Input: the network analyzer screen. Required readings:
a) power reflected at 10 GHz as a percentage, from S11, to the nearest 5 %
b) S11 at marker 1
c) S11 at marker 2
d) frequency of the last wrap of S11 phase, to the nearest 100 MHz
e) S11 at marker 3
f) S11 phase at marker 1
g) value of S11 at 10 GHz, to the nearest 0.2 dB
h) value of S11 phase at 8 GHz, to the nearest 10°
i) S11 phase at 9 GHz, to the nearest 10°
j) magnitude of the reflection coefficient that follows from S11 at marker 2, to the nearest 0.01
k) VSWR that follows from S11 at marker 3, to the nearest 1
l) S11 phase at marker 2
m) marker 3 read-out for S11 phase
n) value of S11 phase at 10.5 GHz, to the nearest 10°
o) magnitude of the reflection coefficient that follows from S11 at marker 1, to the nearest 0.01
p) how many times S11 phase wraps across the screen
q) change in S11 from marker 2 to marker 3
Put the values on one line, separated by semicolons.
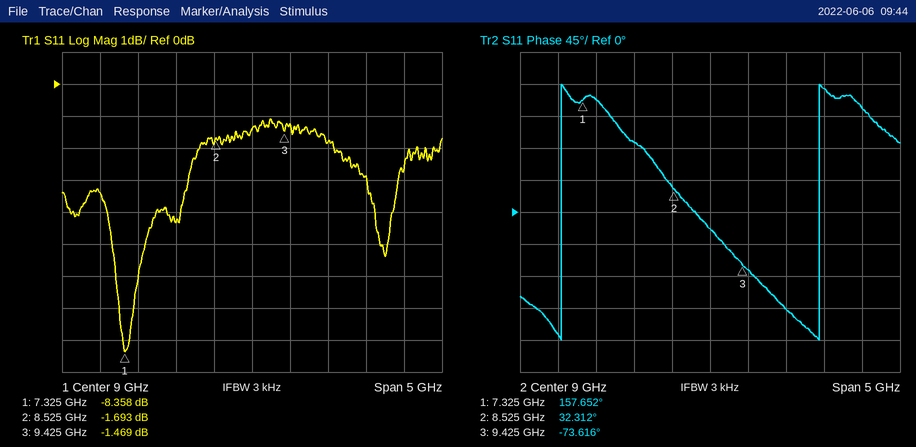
65 %; -8.358 dB; -1.693 dB; 10.4 GHz; -1.469 dB; 157.652°; -1.8 dB; 100°; -20°; 0.82; 12; 32.312°; -73.616°; 170°; 0.38; 2; 0.224 dB
